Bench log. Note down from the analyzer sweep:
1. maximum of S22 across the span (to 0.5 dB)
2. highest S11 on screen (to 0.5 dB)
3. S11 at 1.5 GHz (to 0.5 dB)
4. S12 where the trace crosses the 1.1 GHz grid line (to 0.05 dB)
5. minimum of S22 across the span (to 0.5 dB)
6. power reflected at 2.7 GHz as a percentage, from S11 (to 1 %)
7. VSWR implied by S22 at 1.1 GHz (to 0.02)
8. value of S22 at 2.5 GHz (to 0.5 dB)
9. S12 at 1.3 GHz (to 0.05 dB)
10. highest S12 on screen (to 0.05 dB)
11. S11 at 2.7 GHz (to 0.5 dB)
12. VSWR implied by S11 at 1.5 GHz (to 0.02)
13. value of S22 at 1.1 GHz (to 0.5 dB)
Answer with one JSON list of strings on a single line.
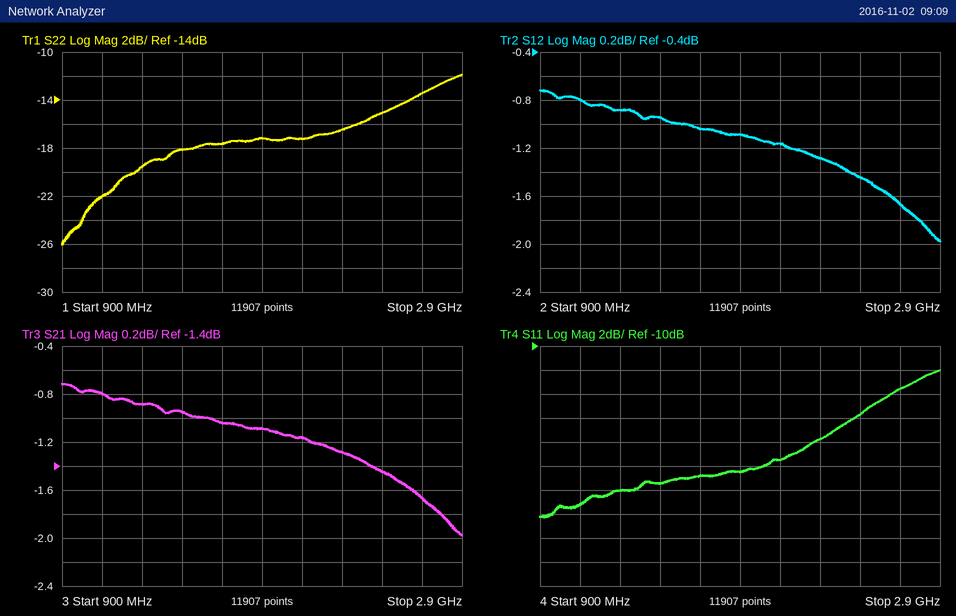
["-12.0 dB", "-12.0 dB", "-21.5 dB", "-0.80 dB", "-26.0 dB", "4 %", "1.18", "-15.0 dB", "-0.90 dB", "-0.70 dB", "-13.5 dB", "1.18", "-22.0 dB"]
